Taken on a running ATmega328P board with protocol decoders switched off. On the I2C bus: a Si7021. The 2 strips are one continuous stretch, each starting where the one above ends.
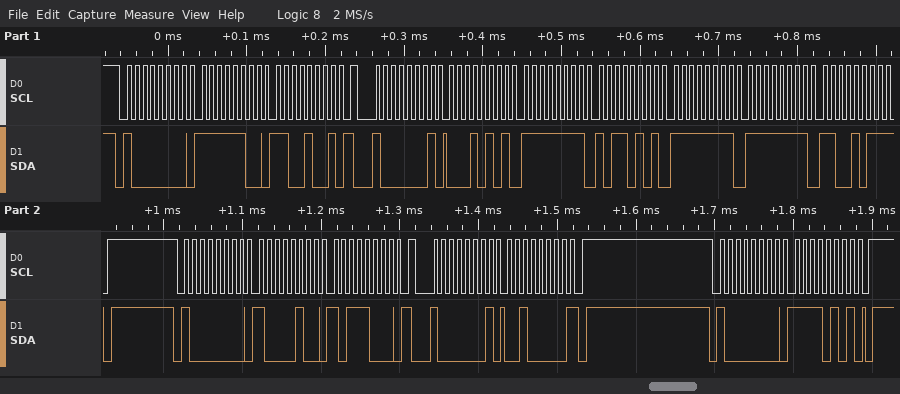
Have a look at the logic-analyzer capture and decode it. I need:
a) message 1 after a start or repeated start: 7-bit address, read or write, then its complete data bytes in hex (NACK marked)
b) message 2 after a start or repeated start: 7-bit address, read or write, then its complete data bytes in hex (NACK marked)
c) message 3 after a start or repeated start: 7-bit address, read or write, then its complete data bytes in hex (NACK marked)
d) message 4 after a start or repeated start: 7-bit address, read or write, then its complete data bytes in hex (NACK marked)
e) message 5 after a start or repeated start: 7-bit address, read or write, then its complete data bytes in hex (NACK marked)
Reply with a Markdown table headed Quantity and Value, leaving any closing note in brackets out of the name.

| Quantity | Value |
|---|---|
| message 1 after a start or repeated start: 7-bit address, read or write, then its complete data bytes in hex | 0x40 write: FC C9 |
| message 2 after a start or repeated start: 7-bit address, read or write, then its complete data bytes in hex | 0x40 read: 15 FF B5 FF FF CB NACK |
| message 3 after a start or repeated start: 7-bit address, read or write, then its complete data bytes in hex | 0x40 write: 84 B8 |
| message 4 after a start or repeated start: 7-bit address, read or write, then its complete data bytes in hex | 0x40 read: 20 NACK |
| message 5 after a start or repeated start: 7-bit address, read or write, then its complete data bytes in hex | 0x40 write: F5 |
